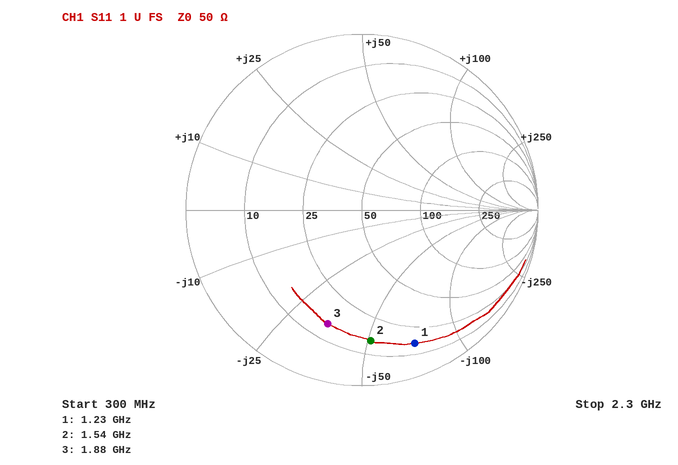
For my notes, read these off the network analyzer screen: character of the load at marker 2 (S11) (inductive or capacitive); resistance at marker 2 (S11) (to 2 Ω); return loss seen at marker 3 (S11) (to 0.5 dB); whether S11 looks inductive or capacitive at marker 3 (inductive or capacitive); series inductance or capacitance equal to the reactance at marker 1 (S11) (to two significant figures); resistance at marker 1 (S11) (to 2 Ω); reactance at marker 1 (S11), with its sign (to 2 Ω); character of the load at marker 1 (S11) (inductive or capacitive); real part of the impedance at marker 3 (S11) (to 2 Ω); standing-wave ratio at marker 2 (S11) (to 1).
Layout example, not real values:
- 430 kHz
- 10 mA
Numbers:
- capacitive
- 16 Ω
- 3.5 dB
- capacitive
- 1.8 pF
- 16 Ω
- -72 Ω
- capacitive
- 14 Ω
- 7
